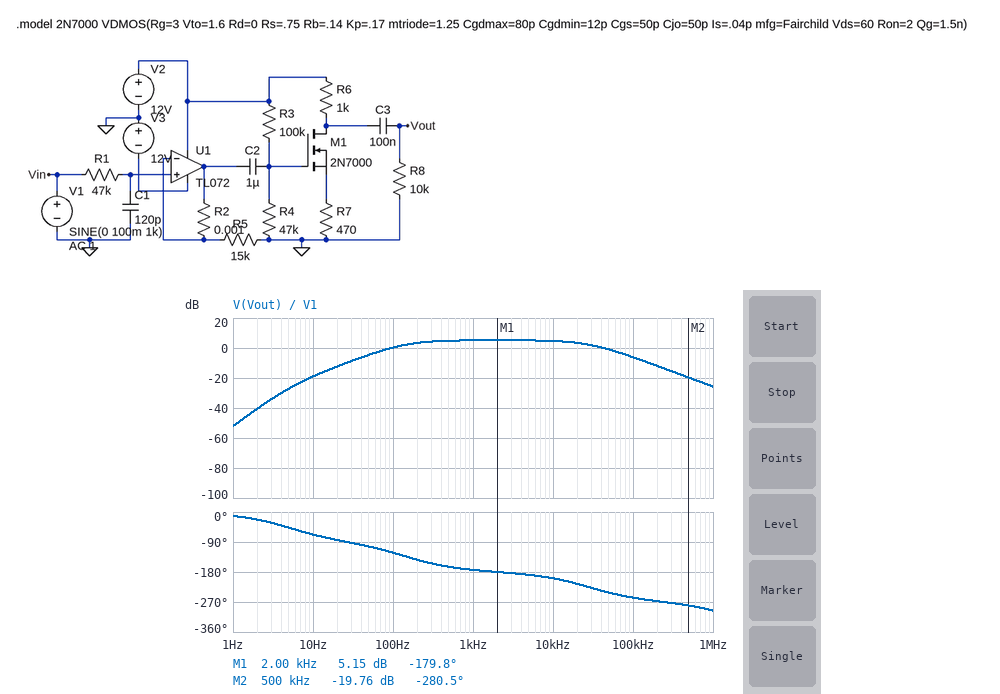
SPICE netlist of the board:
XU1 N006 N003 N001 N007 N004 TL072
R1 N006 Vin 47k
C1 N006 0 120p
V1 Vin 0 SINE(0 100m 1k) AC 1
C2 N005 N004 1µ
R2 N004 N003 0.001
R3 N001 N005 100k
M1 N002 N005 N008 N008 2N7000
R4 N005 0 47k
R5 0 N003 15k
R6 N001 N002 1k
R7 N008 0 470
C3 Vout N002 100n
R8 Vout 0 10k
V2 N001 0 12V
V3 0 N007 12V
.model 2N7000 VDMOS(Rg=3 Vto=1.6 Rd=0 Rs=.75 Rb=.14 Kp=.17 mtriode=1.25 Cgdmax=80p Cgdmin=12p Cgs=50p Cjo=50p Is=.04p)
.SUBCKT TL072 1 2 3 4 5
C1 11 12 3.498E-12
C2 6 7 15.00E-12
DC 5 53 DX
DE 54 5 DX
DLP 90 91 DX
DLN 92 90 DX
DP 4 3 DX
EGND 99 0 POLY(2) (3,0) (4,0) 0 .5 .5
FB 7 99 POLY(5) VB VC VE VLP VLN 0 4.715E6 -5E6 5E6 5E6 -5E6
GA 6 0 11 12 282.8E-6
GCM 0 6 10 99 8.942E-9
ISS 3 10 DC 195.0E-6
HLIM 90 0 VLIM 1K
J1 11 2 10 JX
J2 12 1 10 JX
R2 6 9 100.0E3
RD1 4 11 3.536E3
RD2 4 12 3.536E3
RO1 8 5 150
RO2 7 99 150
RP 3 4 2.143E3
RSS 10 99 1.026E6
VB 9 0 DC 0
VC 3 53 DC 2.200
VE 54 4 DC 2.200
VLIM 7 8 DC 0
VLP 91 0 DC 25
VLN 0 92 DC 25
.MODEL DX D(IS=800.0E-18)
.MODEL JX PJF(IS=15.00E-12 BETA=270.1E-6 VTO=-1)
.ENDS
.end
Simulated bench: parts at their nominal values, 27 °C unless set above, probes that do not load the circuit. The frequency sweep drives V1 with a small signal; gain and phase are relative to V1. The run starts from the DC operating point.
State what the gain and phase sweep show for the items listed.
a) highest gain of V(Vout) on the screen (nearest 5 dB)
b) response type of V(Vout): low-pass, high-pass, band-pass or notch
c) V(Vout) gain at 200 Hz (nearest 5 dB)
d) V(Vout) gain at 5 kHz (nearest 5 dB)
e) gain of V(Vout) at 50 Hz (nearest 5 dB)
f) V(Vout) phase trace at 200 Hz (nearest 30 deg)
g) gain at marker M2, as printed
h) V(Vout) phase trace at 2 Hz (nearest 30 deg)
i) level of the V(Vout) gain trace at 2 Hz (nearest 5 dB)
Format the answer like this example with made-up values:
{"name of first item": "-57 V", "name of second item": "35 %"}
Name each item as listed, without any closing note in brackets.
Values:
{"highest gain of V(Vout) on the screen": "5 dB", "response type of V(Vout): low-pass, high-pass, band-pass or notch": "band-pass", "V(Vout) gain at 200 Hz": "5 dB", "V(Vout) gain at 5 kHz": "5 dB", "gain of V(Vout) at 50 Hz": "-5 dB", "V(Vout) phase trace at 200 Hz": "-150 deg", "gain at marker M2, as printed": "-19.76 dB", "V(Vout) phase trace at 2 Hz": "-30 deg", "level of the V(Vout) gain trace at 2 Hz": "-40 dB"}
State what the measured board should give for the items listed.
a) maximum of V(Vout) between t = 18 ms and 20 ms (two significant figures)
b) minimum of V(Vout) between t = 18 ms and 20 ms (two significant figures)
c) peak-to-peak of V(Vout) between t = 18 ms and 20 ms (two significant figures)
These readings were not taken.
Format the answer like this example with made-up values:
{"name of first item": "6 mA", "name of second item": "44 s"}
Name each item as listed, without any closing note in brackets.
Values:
{"maximum of V(Vout) between t = 18 ms and 20 ms": "180 mV", "minimum of V(Vout) between t = 18 ms and 20 ms": "-180 mV", "peak-to-peak of V(Vout) between t = 18 ms and 20 ms": "360 mV"}
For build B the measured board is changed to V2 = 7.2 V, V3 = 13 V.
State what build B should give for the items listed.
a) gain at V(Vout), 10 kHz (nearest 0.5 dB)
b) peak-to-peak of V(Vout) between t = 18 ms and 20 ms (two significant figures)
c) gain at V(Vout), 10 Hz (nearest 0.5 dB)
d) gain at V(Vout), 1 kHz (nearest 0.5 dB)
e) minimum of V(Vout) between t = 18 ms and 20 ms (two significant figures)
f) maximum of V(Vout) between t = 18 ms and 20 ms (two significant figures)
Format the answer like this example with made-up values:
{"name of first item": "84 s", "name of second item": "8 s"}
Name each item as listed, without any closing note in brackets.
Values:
{"gain at V(Vout), 10 kHz": "4.0 dB", "peak-to-peak of V(Vout) between t = 18 ms and 20 ms": "330 mV", "gain at V(Vout), 10 Hz": "-19.5 dB", "gain at V(Vout), 1 kHz": "4.5 dB", "minimum of V(Vout) between t = 18 ms and 20 ms": "-170 mV", "maximum of V(Vout) between t = 18 ms and 20 ms": "170 mV"}
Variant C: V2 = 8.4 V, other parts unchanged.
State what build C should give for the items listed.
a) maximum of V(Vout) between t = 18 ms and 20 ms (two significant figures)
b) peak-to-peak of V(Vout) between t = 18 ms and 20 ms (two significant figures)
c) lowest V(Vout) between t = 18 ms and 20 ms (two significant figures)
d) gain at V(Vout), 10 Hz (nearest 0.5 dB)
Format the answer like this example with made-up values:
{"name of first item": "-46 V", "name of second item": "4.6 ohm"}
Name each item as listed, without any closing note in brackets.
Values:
{"maximum of V(Vout) between t = 18 ms and 20 ms": "170 mV", "peak-to-peak of V(Vout) between t = 18 ms and 20 ms": "350 mV", "lowest V(Vout) between t = 18 ms and 20 ms": "-170 mV", "gain at V(Vout), 10 Hz": "-19.5 dB"}
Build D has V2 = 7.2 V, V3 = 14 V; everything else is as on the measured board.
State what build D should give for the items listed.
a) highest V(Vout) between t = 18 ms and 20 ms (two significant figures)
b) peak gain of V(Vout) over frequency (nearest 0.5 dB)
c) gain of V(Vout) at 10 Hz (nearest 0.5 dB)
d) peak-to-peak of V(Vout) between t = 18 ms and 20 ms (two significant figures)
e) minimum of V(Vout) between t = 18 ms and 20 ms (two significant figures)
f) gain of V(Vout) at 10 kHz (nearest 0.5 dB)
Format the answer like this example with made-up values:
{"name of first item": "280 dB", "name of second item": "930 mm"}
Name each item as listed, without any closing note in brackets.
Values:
{"highest V(Vout) between t = 18 ms and 20 ms": "170 mV", "peak gain of V(Vout) over frequency": "4.5 dB", "gain of V(Vout) at 10 Hz": "-19.5 dB", "peak-to-peak of V(Vout) between t = 18 ms and 20 ms": "330 mV", "minimum of V(Vout) between t = 18 ms and 20 ms": "-170 mV", "gain of V(Vout) at 10 kHz": "4.0 dB"}
